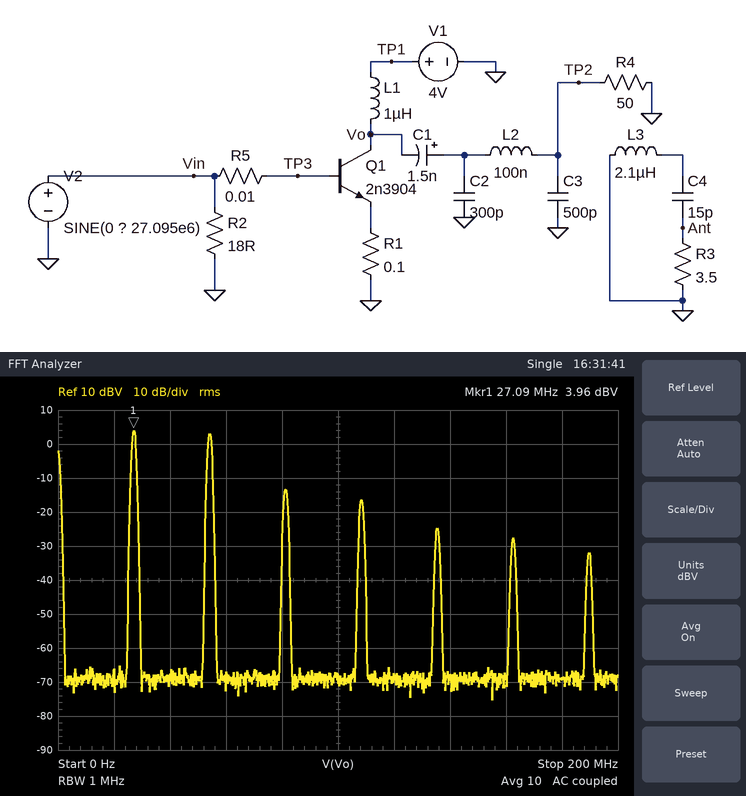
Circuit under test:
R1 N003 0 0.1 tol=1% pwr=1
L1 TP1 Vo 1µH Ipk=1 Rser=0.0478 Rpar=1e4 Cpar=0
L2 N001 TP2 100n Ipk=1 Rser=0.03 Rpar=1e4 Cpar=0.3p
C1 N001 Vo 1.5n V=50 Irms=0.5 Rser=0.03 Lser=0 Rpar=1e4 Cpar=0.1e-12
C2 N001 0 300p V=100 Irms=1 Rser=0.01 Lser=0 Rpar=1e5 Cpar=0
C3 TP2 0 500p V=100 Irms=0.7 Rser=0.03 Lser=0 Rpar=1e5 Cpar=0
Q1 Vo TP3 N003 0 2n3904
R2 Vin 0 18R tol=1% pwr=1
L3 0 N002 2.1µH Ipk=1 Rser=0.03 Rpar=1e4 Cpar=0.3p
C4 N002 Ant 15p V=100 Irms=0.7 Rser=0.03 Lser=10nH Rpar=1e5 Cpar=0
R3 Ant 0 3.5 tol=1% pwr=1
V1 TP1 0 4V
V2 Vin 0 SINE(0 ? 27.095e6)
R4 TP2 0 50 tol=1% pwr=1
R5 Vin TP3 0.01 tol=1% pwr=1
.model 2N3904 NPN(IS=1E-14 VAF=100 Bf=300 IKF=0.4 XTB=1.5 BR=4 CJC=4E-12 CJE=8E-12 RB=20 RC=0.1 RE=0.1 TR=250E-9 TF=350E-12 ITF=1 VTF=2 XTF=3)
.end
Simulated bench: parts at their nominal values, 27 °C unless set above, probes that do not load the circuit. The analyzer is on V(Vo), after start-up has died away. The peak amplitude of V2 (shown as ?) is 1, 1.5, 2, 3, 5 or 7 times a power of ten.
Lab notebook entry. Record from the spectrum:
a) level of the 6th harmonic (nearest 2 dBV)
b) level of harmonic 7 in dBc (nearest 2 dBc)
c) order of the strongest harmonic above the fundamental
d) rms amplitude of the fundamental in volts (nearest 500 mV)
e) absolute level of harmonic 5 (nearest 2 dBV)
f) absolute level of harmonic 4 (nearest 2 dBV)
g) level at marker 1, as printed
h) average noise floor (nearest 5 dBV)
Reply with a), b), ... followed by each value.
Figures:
a) -28 dBV
b) -36 dBc
c) 2
d) 1.5 V
e) -24 dBV
f) -16 dBV
g) 3.96 dBV
h) -70 dBV
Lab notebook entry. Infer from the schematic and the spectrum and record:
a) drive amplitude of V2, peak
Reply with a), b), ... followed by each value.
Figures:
a) 2 V
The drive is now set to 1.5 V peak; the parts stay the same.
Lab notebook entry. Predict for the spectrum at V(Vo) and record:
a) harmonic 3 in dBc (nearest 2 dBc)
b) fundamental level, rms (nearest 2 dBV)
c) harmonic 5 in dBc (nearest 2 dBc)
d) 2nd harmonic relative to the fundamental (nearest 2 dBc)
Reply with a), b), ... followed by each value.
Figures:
a) -20 dBc
b) 0 dBV
c) -26 dBc
d) 2 dBc
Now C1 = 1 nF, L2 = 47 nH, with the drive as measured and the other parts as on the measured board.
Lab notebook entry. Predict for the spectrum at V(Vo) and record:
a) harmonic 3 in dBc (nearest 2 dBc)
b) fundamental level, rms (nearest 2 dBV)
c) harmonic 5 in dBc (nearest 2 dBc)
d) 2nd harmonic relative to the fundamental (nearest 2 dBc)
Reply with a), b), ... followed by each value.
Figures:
a) -6 dBc
b) 6 dBV
c) -28 dBc
d) 4 dBc
